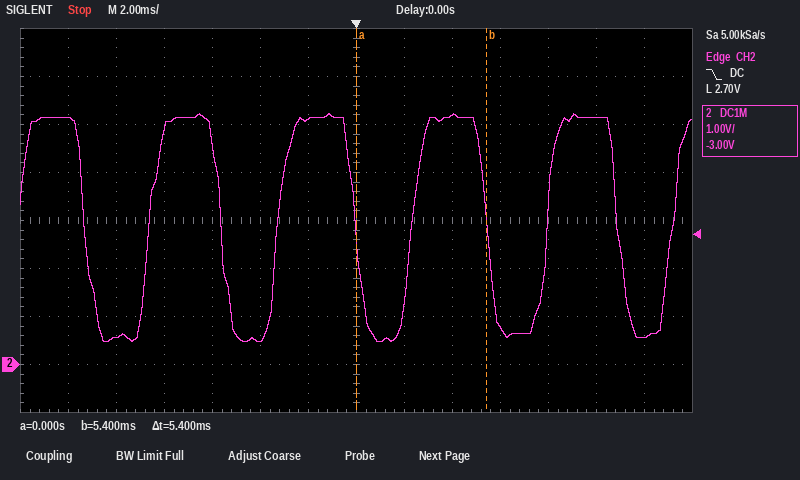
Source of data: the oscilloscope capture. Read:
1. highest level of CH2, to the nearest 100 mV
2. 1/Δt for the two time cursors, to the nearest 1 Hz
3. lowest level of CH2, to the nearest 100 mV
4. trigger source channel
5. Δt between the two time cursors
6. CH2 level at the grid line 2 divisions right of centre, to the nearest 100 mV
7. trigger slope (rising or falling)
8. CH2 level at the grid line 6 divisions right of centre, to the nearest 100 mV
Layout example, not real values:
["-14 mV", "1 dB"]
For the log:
["5.2 V", "185 Hz", "500 mV", "CH2", "5.4 ms", "5.2 V", "falling", "600 mV"]
